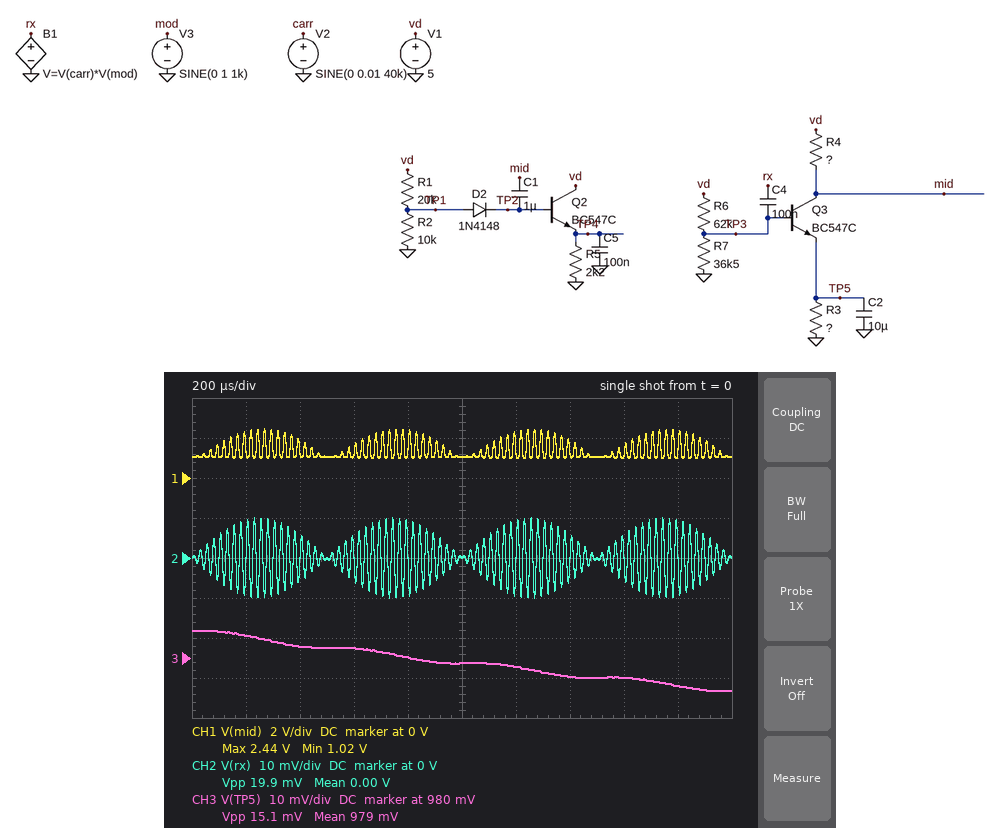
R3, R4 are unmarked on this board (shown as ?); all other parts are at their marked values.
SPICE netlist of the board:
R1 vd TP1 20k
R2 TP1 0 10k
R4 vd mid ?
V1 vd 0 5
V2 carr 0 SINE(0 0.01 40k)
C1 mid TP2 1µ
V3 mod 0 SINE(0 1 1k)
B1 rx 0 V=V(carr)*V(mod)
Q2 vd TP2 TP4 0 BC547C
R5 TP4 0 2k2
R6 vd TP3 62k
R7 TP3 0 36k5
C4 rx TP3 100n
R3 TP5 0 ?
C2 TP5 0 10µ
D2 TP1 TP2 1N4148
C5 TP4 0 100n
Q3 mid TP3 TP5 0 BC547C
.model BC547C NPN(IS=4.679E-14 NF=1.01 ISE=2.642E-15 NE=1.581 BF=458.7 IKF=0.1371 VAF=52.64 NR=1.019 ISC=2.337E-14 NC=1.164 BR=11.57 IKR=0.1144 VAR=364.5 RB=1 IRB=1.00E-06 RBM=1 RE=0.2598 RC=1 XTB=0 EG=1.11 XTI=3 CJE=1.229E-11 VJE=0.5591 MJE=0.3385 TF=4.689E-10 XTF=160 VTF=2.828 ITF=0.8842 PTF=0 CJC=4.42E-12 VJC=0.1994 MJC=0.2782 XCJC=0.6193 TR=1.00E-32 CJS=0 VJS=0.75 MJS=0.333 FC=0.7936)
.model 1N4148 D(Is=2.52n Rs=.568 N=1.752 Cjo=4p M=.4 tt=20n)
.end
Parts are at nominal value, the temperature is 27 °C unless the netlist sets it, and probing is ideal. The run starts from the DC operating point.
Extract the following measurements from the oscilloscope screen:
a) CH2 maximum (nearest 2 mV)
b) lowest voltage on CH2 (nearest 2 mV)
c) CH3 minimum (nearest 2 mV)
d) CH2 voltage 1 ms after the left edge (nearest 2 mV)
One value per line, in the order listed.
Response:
10 mV
-10 mV
972 mV
0 V
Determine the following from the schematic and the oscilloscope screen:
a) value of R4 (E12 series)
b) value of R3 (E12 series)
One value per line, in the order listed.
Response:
3.3 kΩ
820 Ω
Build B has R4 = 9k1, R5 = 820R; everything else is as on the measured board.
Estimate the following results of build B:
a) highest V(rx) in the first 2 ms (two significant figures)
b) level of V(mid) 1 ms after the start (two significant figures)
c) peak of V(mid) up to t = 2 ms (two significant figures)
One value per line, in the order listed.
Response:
10 mV
460 mV
500 mV
